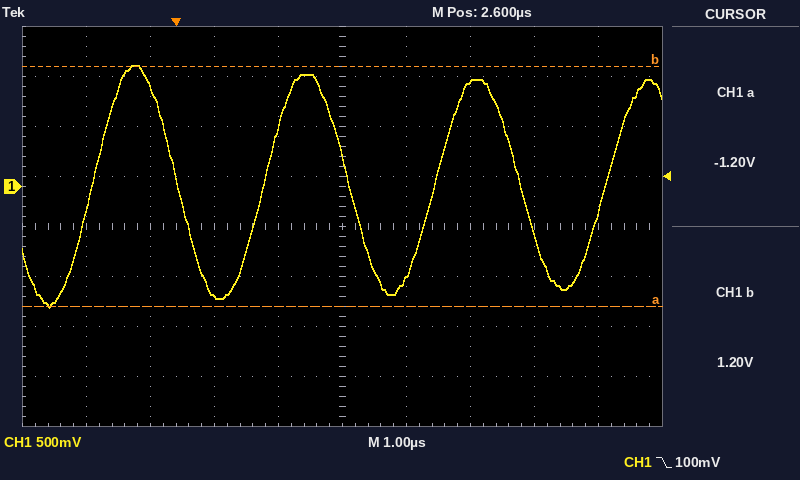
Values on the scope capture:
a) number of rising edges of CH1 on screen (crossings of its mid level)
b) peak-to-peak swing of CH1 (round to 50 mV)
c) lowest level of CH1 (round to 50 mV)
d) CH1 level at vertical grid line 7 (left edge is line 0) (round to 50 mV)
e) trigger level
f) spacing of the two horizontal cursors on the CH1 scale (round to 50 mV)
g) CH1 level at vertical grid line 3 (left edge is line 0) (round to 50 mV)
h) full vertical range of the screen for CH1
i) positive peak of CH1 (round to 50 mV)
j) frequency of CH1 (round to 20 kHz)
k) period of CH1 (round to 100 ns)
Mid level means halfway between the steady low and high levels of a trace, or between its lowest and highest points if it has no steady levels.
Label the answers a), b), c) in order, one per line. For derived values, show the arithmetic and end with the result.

a) 4
b) 1.20 V − (-1.20 V) = 2.40 V
c) -1.20 V
d) 1.05 V
e) 100 mV
f) 2.40 V
g) -1.10 V
h) 4 V
i) 1.20 V
j) 1 / 2.7 µs ≈ 370 kHz, so 380 kHz to the nearest 20 kHz
k) 2.7 µs
